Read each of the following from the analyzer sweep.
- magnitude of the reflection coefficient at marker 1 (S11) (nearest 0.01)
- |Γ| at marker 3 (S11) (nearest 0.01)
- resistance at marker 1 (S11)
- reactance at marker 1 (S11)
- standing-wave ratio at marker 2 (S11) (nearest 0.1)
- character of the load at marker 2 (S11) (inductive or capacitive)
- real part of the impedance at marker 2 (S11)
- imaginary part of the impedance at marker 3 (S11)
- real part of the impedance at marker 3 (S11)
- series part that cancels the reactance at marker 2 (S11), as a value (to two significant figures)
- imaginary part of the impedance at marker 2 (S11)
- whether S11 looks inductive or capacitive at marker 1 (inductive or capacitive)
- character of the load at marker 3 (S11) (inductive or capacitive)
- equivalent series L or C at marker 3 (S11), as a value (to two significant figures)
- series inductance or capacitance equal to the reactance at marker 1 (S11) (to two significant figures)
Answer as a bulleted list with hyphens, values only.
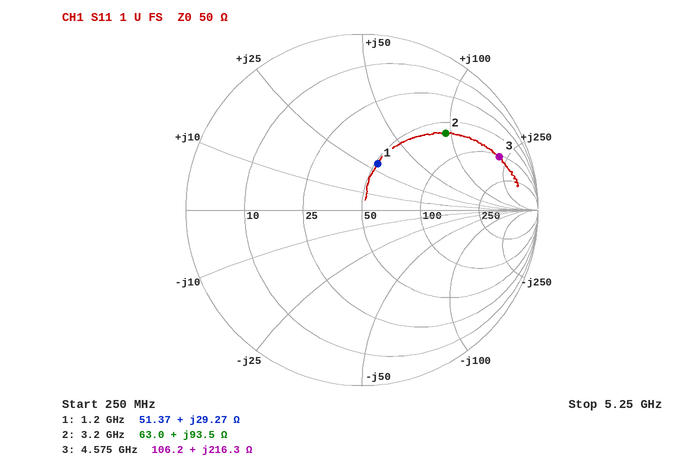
- 0.28
- 0.84
- 51.37 Ω
- +29.27 Ω
- 4.6
- inductive
- 63.0 Ω
- +216.3 Ω
- 106.2 Ω
- 530 fF
- +93.5 Ω
- inductive
- inductive
- 7.5 nH
- 3.9 nH
